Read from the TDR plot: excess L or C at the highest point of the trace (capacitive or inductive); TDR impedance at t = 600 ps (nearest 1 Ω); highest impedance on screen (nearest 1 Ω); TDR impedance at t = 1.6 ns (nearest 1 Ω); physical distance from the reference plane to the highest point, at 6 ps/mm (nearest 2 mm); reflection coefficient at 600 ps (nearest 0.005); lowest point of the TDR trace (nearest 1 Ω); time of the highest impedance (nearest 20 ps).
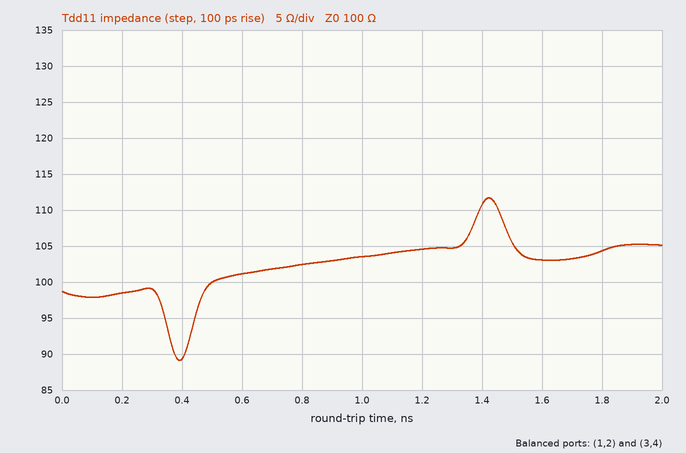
inductive
101 Ω
112 Ω
103 Ω
118 mm
+0.005
89 Ω
1.42 ns
